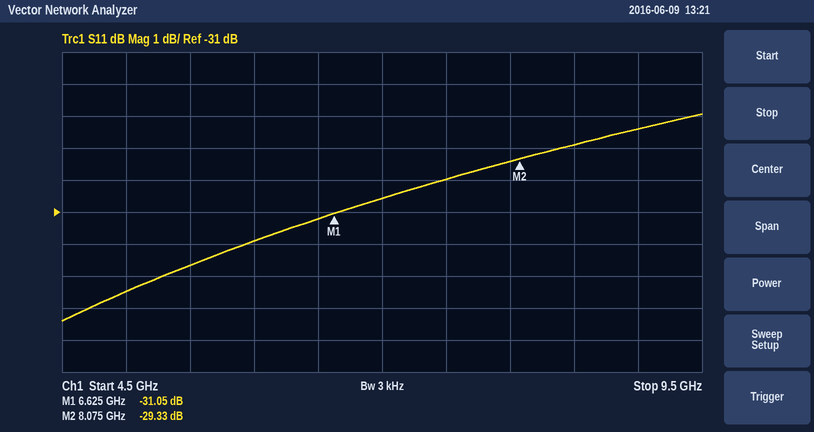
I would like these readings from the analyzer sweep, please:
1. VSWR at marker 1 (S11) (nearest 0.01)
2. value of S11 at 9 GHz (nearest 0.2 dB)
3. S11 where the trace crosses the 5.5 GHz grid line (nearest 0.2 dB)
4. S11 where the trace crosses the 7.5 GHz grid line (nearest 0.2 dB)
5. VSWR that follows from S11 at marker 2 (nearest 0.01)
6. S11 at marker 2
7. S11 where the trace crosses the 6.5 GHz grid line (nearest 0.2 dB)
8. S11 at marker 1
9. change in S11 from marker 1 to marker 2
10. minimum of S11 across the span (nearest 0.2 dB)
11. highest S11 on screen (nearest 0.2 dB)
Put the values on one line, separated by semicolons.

1.06; -28.4 dB; -32.6 dB; -30.0 dB; 1.07; -29.33 dB; -31.2 dB; -31.05 dB; 1.72 dB; -34.4 dB; -28.0 dB
